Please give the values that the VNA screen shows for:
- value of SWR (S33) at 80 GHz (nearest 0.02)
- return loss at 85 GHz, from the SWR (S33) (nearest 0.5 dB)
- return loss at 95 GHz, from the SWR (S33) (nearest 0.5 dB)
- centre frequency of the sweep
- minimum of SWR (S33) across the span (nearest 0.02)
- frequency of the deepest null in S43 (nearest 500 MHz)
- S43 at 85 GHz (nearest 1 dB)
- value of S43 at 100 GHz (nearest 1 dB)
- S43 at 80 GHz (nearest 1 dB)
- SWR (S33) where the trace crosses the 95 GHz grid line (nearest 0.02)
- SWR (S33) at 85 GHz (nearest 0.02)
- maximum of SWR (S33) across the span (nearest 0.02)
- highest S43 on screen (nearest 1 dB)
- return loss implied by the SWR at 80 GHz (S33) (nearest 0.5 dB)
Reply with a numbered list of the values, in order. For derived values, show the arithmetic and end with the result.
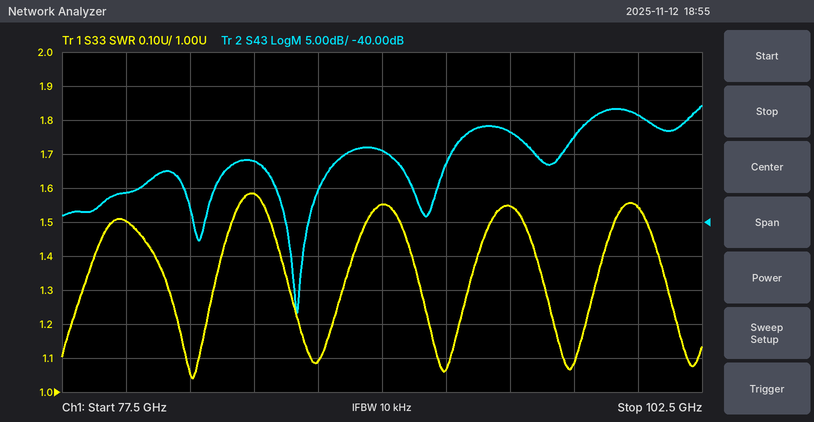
1. 1.50
2. −20 log10((1.58 − 1)/(1.58 + 1)) ≈ 13.0 dB
3. −20 log10((1.54 − 1)/(1.54 + 1)) ≈ 13.4 dB, so 13.5 dB to the nearest 0.5 dB
4. 90 GHz
5. 1.04
6. 86.5 GHz
7. -31 dB
8. -24 dB
9. -36 dB
10. 1.54
11. 1.58
12. 1.58
13. -23 dB
14. −20 log10((1.5 − 1)/(1.5 + 1)) ≈ 14.0 dB
